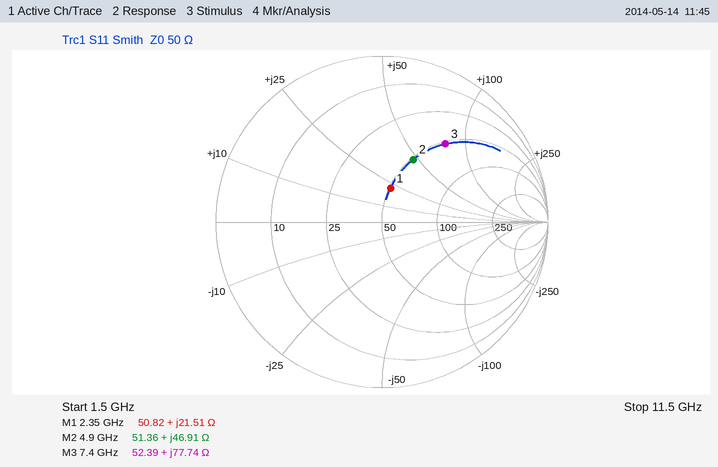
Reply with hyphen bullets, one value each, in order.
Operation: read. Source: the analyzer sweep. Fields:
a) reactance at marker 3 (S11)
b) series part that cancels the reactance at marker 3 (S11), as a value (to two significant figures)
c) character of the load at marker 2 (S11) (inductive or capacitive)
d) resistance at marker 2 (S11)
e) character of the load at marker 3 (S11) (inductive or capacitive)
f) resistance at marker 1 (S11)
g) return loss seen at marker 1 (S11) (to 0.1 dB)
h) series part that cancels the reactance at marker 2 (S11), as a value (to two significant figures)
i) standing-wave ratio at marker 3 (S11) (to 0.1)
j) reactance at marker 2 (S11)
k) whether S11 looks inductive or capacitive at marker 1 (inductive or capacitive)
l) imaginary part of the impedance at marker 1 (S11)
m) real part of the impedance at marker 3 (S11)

- +77.74 Ω
- 280 fF
- inductive
- 51.36 Ω
- inductive
- 50.82 Ω
- 13.6 dB
- 690 fF
- 4.1
- +46.91 Ω
- inductive
- +21.51 Ω
- 52.39 Ω
